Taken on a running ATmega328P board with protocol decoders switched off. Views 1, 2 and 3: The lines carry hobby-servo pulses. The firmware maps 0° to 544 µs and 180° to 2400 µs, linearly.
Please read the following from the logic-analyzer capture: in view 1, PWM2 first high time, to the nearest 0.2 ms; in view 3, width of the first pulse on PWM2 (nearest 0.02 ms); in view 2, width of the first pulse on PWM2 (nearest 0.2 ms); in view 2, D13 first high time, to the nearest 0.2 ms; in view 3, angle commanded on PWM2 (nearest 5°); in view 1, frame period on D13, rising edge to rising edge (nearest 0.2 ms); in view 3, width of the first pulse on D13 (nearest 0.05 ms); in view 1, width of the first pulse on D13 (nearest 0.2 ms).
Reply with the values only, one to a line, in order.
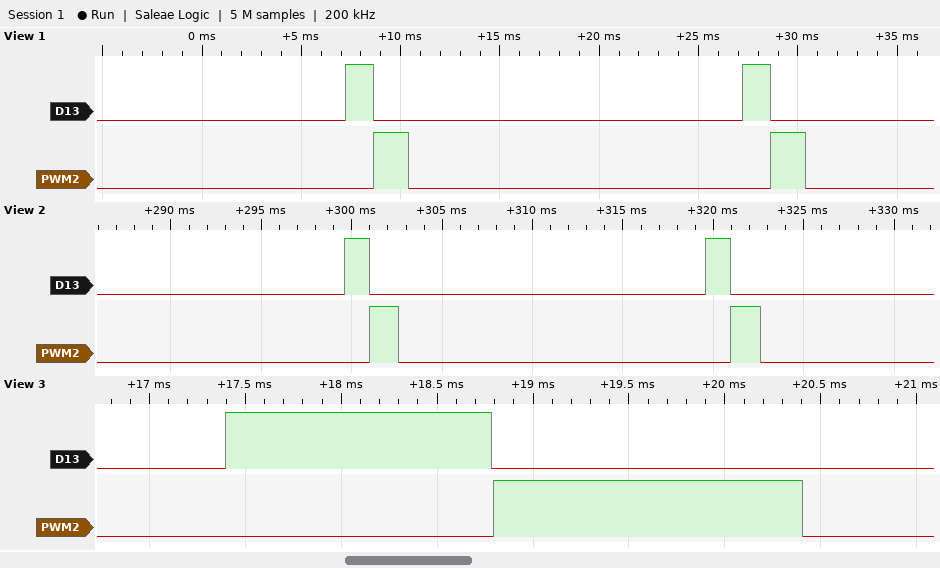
1.8 ms
1.62 ms
1.6 ms
1.4 ms
105°
20.0 ms
1.40 ms
1.4 ms
